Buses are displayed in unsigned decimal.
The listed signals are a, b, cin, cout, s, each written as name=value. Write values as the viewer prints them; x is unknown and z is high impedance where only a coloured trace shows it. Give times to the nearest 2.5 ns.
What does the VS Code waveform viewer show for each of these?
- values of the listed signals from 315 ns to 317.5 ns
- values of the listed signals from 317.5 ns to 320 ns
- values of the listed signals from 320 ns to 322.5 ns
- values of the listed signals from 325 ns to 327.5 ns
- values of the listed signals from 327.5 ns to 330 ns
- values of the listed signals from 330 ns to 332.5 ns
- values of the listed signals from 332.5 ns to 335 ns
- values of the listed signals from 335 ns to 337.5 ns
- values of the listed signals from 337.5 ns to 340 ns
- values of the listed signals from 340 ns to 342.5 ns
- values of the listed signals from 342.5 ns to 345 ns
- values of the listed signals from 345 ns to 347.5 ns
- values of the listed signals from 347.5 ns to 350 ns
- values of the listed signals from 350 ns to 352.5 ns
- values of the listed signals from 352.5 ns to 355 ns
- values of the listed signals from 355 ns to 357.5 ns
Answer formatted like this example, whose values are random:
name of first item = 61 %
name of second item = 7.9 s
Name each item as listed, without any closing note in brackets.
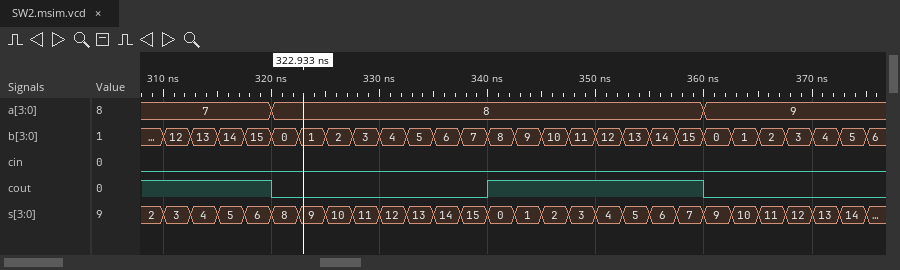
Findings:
values of the listed signals from 315 ns to 317.5 ns = a=7, b=14, cin=0, cout=1, s=5
values of the listed signals from 317.5 ns to 320 ns = a=7, b=15, cin=0, cout=1, s=6
values of the listed signals from 320 ns to 322.5 ns = a=8, b=0, cin=0, cout=0, s=8
values of the listed signals from 325 ns to 327.5 ns = a=8, b=2, cin=0, cout=0, s=10
values of the listed signals from 327.5 ns to 330 ns = a=8, b=3, cin=0, cout=0, s=11
values of the listed signals from 330 ns to 332.5 ns = a=8, b=4, cin=0, cout=0, s=12
values of the listed signals from 332.5 ns to 335 ns = a=8, b=5, cin=0, cout=0, s=13
values of the listed signals from 335 ns to 337.5 ns = a=8, b=6, cin=0, cout=0, s=14
values of the listed signals from 337.5 ns to 340 ns = a=8, b=7, cin=0, cout=0, s=15
values of the listed signals from 340 ns to 342.5 ns = a=8, b=8, cin=0, cout=1, s=0
values of the listed signals from 342.5 ns to 345 ns = a=8, b=9, cin=0, cout=1, s=1
values of the listed signals from 345 ns to 347.5 ns = a=8, b=10, cin=0, cout=1, s=2
values of the listed signals from 347.5 ns to 350 ns = a=8, b=11, cin=0, cout=1, s=3
values of the listed signals from 350 ns to 352.5 ns = a=8, b=12, cin=0, cout=1, s=4
values of the listed signals from 352.5 ns to 355 ns = a=8, b=13, cin=0, cout=1, s=5
values of the listed signals from 355 ns to 357.5 ns = a=8, b=14, cin=0, cout=1, s=6
